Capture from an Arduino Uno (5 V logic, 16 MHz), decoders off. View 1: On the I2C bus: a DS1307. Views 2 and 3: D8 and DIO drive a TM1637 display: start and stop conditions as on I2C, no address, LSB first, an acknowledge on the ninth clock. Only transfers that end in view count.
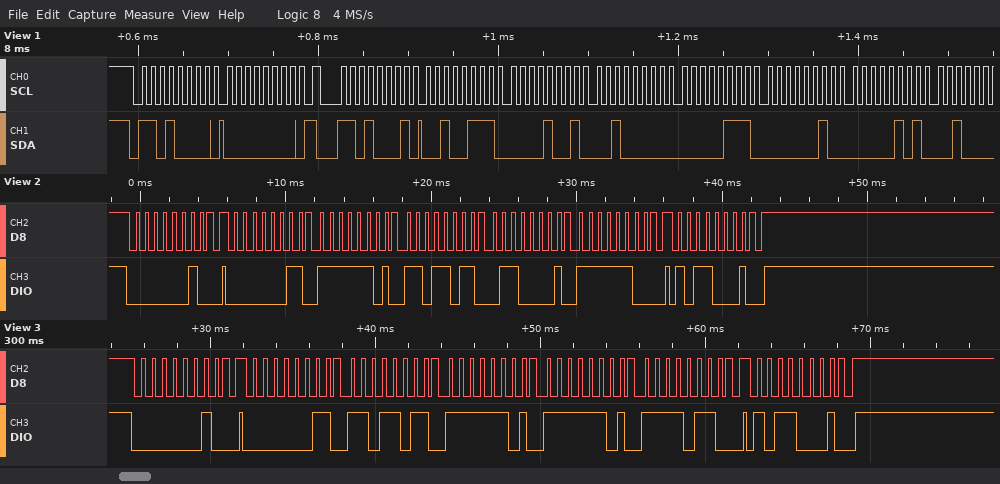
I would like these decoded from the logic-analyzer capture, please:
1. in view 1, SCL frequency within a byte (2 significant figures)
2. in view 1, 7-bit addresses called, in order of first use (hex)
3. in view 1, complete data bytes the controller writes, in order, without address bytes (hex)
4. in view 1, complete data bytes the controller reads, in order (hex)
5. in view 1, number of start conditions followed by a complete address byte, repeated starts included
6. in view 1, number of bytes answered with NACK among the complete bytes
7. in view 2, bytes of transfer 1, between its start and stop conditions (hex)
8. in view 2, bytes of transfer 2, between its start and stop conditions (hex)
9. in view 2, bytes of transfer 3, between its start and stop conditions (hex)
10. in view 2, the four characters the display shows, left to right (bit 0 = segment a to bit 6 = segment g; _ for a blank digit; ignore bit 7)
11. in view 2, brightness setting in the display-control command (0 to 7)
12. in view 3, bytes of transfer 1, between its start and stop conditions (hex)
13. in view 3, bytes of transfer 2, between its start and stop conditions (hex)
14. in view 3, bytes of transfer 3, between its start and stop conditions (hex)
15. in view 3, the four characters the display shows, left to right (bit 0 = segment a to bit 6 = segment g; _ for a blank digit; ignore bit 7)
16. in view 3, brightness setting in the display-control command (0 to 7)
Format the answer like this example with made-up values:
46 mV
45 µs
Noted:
100 kHz
0x68
00
27 09 20 07 02 05
2
0
40
C0 BF DB 86 3F
8D
0210
5
40
C0 DB BF BF 6F
8D
2009
5
